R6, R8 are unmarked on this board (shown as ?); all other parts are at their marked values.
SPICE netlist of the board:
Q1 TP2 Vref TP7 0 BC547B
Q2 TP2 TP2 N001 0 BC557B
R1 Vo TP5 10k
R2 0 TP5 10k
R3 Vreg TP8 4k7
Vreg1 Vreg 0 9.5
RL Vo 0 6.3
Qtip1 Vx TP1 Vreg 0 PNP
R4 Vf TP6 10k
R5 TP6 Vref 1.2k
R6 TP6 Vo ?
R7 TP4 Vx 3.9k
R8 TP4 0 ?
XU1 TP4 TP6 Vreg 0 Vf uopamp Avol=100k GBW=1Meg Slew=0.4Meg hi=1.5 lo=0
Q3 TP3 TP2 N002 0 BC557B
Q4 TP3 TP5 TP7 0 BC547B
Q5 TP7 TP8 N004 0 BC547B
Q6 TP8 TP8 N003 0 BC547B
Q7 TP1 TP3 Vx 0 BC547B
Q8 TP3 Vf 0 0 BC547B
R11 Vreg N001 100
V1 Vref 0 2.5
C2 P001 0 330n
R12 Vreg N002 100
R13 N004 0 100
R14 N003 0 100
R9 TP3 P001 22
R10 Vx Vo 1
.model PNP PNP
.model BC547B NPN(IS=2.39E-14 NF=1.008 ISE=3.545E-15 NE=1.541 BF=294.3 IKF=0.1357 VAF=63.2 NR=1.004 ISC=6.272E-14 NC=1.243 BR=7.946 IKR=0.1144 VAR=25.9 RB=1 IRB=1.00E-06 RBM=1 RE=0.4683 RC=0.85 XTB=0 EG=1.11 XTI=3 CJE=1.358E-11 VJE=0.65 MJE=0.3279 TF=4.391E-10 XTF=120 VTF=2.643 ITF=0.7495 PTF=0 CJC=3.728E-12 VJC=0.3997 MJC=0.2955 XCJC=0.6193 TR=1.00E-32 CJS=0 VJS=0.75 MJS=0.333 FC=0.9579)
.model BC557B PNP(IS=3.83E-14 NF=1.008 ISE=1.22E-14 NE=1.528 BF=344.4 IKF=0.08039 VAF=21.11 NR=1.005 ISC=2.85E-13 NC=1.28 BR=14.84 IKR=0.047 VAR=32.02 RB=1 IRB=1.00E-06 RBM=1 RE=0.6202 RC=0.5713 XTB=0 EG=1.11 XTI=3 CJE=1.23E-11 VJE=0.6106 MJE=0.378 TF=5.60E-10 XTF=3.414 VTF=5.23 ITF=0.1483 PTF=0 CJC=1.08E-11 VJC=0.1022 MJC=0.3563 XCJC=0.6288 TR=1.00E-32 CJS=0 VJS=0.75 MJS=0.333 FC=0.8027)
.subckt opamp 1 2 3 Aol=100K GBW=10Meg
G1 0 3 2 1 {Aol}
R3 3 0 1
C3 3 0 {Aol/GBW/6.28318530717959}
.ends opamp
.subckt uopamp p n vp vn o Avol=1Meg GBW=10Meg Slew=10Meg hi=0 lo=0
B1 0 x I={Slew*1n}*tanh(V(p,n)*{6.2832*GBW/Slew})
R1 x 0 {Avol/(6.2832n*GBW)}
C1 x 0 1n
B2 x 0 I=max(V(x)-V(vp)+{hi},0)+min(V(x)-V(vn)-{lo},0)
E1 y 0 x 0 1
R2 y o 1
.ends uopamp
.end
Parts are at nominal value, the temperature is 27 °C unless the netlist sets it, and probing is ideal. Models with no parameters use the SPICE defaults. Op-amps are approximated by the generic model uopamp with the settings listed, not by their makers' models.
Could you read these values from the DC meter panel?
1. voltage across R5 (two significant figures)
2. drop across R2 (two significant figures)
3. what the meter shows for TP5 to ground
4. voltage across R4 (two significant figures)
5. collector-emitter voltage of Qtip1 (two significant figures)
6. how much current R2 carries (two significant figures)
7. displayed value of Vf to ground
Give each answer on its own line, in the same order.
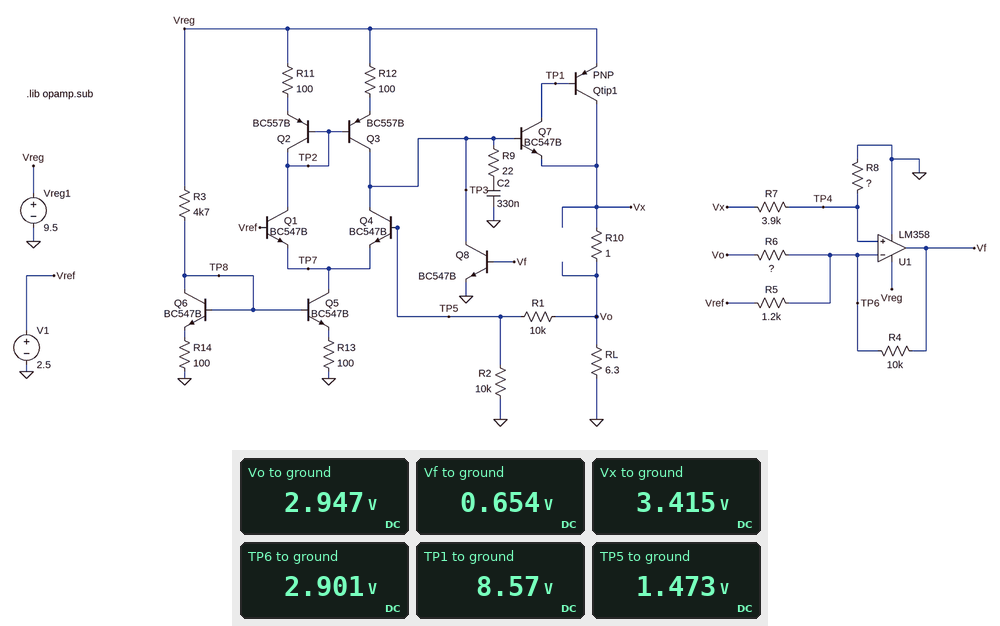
400 mV
1.5 V
1.473 V
2.2 V
-6.1 V
150 µA
0.654 V
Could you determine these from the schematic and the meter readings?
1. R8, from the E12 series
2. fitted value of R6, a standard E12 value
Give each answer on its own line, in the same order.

22 kΩ
82 Ω
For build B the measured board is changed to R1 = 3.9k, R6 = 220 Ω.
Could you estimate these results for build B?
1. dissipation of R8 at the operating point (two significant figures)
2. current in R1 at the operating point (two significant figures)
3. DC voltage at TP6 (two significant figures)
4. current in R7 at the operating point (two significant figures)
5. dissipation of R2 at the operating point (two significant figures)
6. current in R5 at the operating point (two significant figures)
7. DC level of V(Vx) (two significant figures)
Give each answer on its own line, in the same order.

280 µW
180 µA
2.5 V
110 µA
330 µW
4.0 µA
2.9 V
